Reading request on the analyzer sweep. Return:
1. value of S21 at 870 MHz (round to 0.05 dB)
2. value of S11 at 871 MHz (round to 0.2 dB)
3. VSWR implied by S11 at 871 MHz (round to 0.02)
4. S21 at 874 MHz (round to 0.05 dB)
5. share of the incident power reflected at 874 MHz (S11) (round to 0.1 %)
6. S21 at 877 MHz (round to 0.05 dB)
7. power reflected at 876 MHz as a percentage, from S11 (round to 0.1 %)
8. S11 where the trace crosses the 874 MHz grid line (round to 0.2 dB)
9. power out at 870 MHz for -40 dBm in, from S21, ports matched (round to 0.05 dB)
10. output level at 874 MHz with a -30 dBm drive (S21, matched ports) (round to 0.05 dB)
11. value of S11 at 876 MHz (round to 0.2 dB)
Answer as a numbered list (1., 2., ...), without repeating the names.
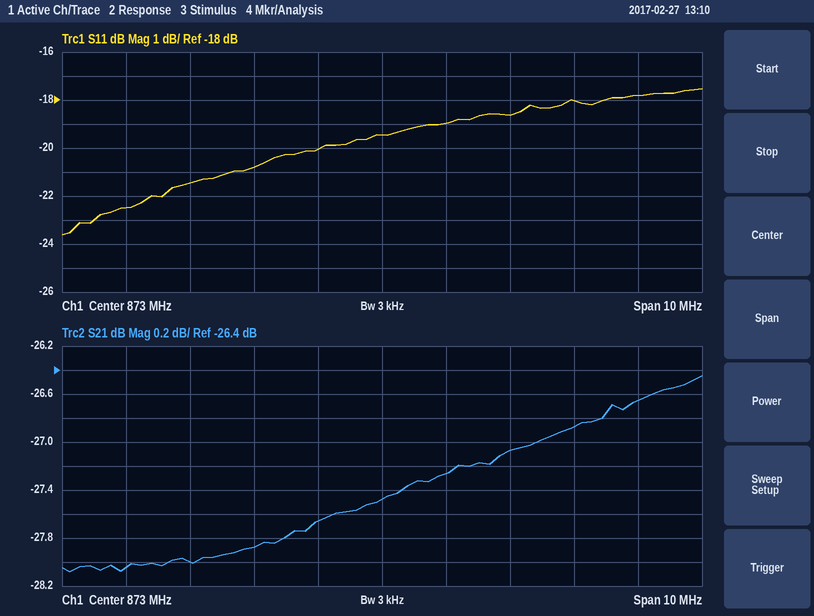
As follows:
1. -28.00 dB
2. -20.8 dB
3. 1.20
4. -27.25 dB
5. 1.3 %
6. -26.65 dB
7. 1.6 %
8. -19.0 dB
9. -68.00 dBm
10. -57.25 dBm
11. -18.0 dB
